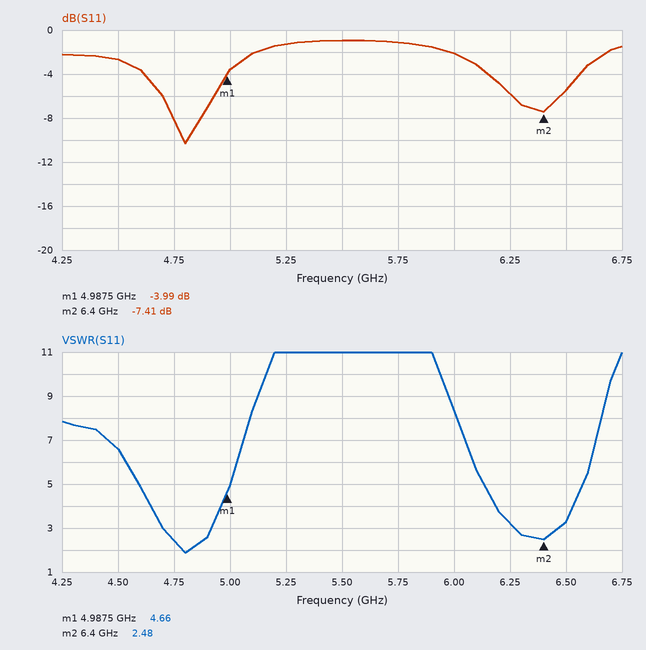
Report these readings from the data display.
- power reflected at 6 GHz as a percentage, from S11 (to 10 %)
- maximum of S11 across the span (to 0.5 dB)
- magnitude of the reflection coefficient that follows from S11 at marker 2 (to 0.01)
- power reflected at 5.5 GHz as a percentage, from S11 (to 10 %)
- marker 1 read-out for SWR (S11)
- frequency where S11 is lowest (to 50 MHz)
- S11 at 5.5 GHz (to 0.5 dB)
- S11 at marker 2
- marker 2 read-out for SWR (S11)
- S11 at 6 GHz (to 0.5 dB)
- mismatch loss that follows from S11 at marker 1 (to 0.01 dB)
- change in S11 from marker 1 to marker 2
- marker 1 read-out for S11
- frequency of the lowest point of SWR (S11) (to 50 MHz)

60 %
-1.0 dB
0.43
80 %
4.66
4.80 GHz
-1.0 dB
-7.41 dB
2.48
-2.0 dB
2.21 dB
-3.42 dB
-3.99 dB
4.80 GHz
